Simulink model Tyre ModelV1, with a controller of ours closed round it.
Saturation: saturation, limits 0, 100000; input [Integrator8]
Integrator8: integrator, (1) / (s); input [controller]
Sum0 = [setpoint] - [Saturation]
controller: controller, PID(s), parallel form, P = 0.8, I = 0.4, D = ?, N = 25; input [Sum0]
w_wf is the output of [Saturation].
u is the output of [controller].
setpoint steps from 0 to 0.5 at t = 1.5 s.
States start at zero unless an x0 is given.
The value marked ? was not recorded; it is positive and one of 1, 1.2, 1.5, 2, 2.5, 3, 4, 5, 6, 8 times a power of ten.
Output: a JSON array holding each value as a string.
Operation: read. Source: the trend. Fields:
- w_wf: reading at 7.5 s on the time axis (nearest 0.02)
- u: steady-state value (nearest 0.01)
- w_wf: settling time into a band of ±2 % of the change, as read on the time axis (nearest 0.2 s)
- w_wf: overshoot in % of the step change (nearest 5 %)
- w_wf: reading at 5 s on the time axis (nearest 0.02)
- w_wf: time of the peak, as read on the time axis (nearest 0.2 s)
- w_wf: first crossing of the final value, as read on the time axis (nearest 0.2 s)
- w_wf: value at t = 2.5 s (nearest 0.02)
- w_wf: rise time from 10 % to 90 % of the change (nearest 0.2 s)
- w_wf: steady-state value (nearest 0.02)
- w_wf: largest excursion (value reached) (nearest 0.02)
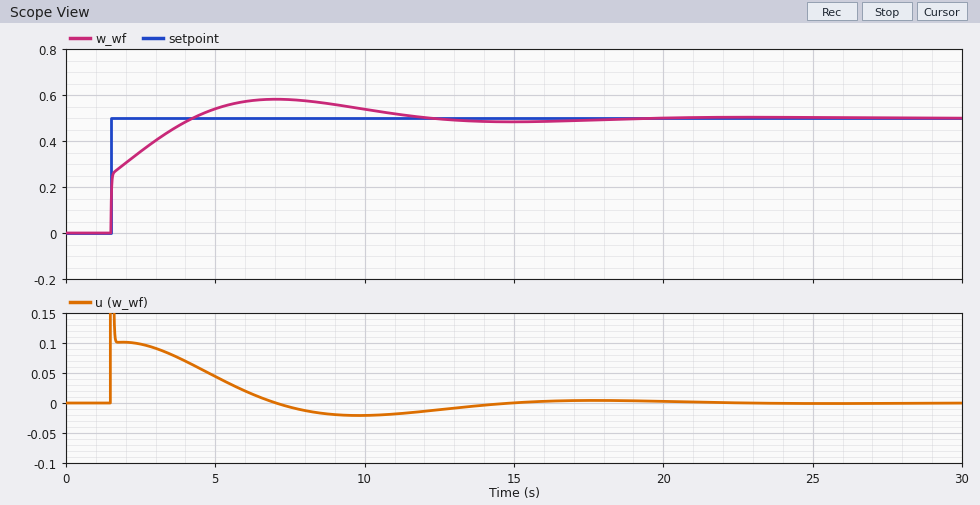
["0.58", "0.00", "17.4 s", "15 %", "0.54", "7.0 s", "4.2 s", "0.36", "2.0 s", "0.50", "0.58"]
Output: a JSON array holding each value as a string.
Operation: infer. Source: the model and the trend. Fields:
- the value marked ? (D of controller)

["1"]
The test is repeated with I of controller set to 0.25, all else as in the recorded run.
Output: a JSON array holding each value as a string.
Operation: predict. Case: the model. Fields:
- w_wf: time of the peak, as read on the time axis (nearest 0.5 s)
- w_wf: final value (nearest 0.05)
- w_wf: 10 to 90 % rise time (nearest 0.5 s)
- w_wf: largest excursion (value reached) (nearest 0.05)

["8.0 s", "0.50", "2.5 s", "0.55"]
